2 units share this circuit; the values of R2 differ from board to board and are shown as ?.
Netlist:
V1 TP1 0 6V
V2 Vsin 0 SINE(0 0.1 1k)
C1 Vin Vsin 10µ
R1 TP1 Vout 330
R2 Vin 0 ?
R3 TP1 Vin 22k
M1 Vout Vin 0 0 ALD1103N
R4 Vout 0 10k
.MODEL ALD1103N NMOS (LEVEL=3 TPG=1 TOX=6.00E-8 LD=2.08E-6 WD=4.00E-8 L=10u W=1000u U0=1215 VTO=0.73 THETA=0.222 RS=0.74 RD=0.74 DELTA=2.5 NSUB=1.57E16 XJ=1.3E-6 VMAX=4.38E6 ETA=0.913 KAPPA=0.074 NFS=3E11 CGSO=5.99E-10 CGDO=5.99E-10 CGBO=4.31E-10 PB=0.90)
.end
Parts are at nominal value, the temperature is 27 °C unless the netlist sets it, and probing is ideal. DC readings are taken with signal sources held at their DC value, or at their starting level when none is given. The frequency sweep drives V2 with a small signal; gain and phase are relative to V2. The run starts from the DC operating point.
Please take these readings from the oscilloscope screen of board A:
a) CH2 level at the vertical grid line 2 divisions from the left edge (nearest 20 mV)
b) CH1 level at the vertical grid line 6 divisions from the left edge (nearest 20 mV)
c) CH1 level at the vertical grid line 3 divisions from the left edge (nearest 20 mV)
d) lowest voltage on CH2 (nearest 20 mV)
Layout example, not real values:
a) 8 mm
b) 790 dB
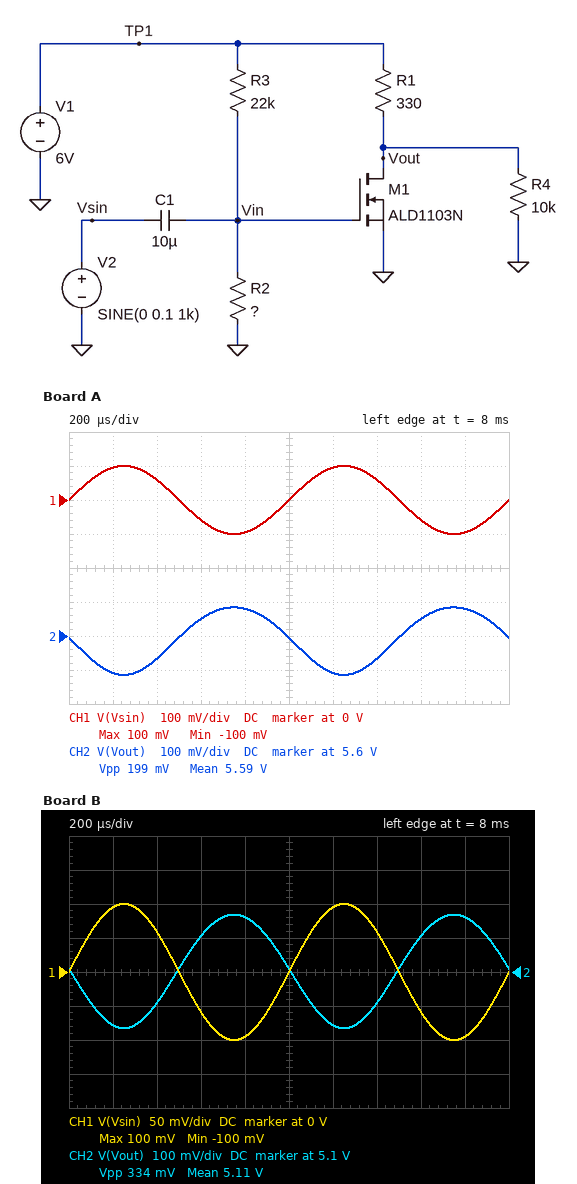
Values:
a) 5.54 V
b) 100 mV
c) -60 mV
d) 5.48 V
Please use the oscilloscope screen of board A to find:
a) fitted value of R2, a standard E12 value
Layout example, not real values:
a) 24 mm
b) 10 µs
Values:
a) 4.7 kΩ
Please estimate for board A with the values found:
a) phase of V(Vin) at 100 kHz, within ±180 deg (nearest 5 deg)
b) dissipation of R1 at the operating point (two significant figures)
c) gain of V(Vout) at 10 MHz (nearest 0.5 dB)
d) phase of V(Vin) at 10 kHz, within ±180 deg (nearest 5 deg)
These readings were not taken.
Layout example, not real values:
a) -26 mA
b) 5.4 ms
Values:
a) 0 deg
b) 500 µW
c) 0 dB
d) 0 deg
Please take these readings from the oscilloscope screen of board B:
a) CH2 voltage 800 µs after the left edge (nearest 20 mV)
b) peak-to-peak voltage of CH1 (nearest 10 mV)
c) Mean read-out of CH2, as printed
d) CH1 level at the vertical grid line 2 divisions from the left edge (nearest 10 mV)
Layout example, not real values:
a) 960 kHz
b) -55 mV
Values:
a) 5.26 V
b) 200 mV
c) 5.11 V
d) 60 mV
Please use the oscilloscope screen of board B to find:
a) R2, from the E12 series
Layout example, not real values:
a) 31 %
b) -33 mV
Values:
a) 6.8 kΩ
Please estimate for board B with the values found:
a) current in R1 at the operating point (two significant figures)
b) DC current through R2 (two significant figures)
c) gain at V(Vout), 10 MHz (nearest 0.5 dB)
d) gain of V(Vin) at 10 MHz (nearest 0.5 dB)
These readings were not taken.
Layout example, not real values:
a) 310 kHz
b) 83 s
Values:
a) 2.7 mA
b) 210 µA
c) 4.5 dB
d) 0 dB
